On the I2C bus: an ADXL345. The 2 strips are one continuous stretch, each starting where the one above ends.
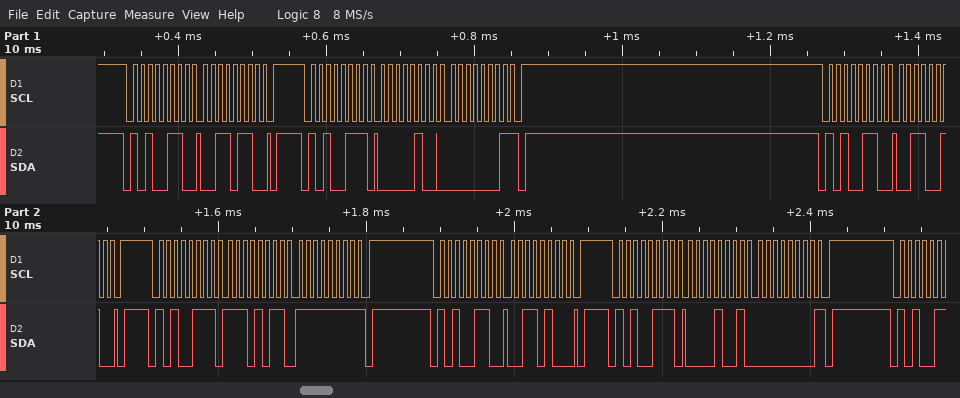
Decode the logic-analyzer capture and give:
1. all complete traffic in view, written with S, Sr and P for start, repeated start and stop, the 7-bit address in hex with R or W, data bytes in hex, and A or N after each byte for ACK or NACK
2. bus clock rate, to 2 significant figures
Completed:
S 53W A 36 A P S 53R A 04 A 01 N P S 53W A 32 A P S 53R A EB A FF N P S 53W A 34 A P S 53R A 09 A 00 N P
100 kHz
